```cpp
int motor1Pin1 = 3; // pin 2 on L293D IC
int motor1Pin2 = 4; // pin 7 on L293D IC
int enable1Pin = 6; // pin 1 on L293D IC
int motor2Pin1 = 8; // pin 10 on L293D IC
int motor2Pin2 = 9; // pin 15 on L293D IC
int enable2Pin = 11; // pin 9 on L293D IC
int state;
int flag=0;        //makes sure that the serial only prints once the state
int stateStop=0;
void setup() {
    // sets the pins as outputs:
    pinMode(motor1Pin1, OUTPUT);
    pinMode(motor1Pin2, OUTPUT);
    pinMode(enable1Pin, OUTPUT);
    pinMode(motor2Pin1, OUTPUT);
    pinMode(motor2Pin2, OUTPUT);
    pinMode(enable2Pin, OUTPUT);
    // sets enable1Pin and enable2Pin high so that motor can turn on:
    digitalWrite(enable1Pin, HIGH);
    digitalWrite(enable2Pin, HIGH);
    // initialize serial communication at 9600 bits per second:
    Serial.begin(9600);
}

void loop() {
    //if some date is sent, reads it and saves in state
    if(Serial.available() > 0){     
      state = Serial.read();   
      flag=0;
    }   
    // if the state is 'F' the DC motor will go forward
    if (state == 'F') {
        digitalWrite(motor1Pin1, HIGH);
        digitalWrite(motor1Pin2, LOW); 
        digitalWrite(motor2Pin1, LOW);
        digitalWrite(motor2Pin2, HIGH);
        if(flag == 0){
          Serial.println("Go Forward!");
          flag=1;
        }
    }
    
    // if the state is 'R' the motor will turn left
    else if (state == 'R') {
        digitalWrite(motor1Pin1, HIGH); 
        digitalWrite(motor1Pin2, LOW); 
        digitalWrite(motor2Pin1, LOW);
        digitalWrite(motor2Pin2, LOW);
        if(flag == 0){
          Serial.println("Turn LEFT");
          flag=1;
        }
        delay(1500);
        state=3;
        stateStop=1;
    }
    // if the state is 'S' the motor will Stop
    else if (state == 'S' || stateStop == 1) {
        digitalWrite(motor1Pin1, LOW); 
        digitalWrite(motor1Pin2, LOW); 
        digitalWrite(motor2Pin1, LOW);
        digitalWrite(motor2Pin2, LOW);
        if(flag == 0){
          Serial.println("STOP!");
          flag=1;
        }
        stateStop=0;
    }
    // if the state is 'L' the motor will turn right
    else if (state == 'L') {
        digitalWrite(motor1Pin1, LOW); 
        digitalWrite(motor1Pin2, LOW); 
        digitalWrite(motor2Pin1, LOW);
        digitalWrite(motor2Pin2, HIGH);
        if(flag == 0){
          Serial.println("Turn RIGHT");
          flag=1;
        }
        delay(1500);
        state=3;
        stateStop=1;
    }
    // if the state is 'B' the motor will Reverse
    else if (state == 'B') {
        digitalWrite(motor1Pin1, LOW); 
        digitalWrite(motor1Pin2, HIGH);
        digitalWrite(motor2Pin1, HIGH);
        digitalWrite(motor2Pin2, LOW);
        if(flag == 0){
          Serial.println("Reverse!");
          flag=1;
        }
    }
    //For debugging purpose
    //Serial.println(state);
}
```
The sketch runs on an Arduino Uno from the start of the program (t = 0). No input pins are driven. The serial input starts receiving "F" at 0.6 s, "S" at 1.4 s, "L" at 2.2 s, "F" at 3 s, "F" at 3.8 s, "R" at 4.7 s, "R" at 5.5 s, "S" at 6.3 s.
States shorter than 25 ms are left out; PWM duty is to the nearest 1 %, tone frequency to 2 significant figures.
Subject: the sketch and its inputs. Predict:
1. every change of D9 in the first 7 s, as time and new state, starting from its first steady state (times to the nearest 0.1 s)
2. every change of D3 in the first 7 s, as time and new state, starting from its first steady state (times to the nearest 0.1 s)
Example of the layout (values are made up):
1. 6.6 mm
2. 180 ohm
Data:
1. 0 s low; 0.6 s high; 1.4 s low; 2.2 s high; 4.7 s low
2. 0 s low; 0.6 s high; 1.4 s low; 3.7 s high
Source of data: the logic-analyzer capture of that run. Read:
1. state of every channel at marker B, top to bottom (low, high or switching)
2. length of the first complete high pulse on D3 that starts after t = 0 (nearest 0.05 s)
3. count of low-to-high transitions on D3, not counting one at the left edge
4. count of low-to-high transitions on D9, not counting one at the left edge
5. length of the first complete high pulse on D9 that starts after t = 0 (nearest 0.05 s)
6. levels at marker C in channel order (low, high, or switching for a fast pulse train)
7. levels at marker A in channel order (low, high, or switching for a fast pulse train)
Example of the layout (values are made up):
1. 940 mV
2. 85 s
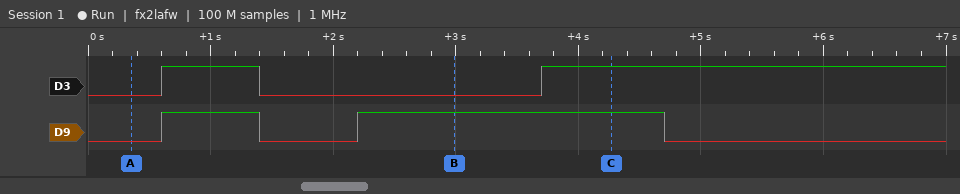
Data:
1. D3 low, D9 high
2. 0.80 s
3. 2
4. 2
5. 0.80 s
6. D3 high, D9 high
7. D3 low, D9 low
